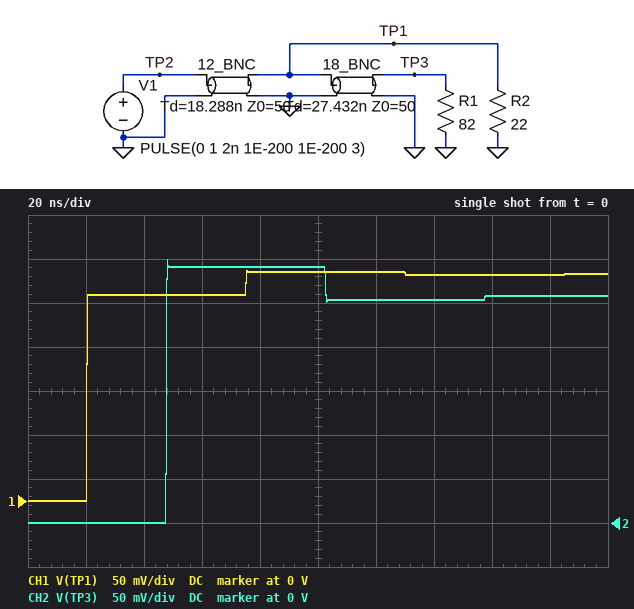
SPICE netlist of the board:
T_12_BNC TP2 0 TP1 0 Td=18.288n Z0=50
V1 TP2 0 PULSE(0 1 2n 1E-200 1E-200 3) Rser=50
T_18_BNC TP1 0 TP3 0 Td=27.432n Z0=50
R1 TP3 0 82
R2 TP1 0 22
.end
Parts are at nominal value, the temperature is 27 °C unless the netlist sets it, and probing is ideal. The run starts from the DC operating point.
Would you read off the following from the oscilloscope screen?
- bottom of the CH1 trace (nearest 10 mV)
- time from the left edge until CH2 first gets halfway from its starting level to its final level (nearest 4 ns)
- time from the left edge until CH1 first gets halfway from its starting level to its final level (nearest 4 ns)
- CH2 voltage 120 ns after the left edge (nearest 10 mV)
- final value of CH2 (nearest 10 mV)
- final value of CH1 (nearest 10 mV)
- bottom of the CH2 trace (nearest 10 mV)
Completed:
0 V
48 ns
20 ns
250 mV
260 mV
260 mV
0 V
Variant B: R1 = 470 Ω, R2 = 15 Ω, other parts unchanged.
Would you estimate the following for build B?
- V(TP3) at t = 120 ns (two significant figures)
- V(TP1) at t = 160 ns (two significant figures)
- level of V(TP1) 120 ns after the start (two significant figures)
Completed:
170 mV
220 mV
240 mV
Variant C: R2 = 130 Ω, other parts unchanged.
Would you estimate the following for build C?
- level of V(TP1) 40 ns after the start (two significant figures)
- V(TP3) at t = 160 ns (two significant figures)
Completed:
420 mV
500 mV
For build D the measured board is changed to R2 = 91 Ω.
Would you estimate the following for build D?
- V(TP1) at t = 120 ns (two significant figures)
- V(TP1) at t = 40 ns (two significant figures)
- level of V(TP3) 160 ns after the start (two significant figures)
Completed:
470 mV
390 mV
460 mV
